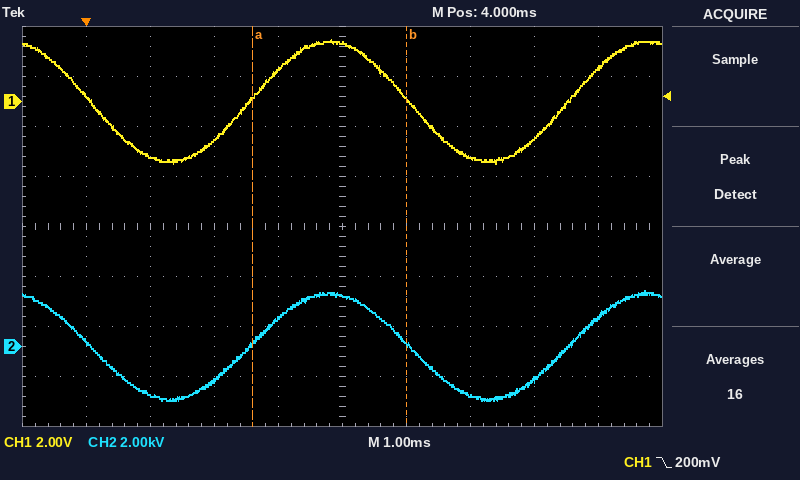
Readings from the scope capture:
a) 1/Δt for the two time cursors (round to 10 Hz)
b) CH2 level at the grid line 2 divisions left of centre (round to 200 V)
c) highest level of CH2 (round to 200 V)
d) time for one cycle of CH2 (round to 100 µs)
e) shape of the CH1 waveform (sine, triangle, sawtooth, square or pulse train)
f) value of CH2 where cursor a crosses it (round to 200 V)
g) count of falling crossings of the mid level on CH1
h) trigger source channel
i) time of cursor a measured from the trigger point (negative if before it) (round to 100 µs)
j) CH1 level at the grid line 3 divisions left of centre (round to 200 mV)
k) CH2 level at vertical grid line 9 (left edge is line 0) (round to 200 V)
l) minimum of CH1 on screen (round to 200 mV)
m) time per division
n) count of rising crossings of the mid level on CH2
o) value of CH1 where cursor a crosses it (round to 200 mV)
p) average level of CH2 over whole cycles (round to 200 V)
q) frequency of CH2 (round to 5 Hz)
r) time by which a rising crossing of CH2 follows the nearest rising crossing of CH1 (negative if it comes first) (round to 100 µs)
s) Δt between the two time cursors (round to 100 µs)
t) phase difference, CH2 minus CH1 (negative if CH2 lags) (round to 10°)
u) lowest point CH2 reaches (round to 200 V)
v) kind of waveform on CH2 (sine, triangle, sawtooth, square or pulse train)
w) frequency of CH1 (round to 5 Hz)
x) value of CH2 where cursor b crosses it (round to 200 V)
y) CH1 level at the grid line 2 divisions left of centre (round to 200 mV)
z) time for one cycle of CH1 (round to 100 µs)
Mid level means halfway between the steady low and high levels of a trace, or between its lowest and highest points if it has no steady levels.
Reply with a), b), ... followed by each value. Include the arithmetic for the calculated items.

a) 1 / 2.4 ms ≈ 420 Hz
b) -1.4 kV
c) 2.2 kV
d) 5.0 ms
e) sine
f) 200 V
g) 2
h) CH1
i) +2.6 ms
j) -2.2 V
k) 1.2 kV
l) -2.4 V
m) 1 ms
n) 2
o) 200 mV
p) (2.2 kV + (-2.2 kV)) / 2 ≈ 0.0 kV
q) 1 / 5.0 ms ≈ 200 Hz
r) 0.0 ms
s) 2.4 ms
t) −360° × (0.0 ms) / 5.0 ms ≈ 0°
u) -2.2 kV
v) sine
w) 1 / 5.0 ms ≈ 200 Hz
x) 200 V
y) -1.6 V
z) 5.0 ms
